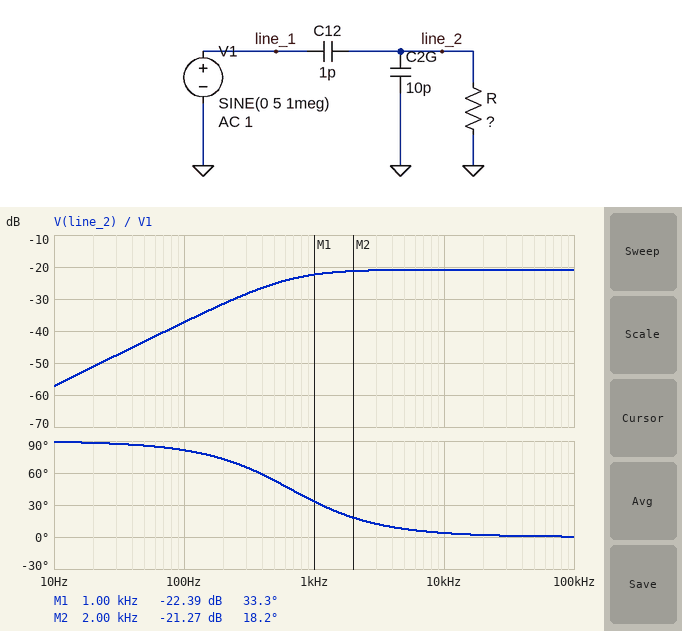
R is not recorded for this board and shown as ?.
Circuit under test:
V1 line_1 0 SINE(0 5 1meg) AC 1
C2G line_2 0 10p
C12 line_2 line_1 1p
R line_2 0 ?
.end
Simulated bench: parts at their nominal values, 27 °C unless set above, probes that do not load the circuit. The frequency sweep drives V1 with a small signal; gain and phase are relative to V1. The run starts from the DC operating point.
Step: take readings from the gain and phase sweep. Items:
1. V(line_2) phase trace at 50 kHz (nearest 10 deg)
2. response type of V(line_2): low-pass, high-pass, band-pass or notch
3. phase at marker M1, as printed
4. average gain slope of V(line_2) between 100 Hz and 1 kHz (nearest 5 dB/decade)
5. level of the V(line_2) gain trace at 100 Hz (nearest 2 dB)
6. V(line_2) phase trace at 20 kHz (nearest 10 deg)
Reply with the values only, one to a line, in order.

0 deg
high-pass
33.3 deg
15 dB/decade
-38 dB
0 deg
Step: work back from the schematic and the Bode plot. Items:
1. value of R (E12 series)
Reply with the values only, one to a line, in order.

22 MΩ
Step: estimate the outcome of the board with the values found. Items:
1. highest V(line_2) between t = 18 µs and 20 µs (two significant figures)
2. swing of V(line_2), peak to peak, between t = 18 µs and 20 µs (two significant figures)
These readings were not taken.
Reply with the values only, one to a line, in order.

450 mV
910 mV
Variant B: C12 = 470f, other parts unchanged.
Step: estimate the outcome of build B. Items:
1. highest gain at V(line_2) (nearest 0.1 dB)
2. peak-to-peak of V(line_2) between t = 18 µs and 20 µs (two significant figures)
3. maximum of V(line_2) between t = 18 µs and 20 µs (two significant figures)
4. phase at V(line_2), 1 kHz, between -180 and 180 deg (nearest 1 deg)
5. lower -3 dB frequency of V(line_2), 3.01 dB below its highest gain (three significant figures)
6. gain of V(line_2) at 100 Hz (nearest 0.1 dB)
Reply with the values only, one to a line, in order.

-27.0 dB
450 mV
220 mV
35 deg
691 Hz
-43.8 dB
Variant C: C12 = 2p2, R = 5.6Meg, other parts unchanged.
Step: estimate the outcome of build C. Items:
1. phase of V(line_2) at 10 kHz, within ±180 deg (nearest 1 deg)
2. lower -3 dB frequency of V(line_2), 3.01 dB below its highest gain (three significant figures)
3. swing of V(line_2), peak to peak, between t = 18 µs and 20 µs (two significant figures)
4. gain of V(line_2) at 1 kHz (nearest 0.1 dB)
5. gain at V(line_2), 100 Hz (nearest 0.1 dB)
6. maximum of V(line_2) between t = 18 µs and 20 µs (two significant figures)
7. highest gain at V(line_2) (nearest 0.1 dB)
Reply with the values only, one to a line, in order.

13 deg
2.33 kHz
1.8 V
-23.0 dB
-42.2 dB
900 mV
-14.9 dB
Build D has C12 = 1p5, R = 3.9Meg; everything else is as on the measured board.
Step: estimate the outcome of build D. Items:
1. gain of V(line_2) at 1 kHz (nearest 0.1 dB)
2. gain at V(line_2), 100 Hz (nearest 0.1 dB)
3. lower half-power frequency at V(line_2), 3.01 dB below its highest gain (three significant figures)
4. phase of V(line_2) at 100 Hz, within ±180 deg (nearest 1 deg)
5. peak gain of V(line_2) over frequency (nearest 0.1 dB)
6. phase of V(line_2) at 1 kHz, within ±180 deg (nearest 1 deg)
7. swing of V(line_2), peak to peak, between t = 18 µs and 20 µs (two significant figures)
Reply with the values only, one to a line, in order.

-29.0 dB
-48.7 dB
3.55 kHz
88 deg
-17.7 dB
74 deg
1.3 V
